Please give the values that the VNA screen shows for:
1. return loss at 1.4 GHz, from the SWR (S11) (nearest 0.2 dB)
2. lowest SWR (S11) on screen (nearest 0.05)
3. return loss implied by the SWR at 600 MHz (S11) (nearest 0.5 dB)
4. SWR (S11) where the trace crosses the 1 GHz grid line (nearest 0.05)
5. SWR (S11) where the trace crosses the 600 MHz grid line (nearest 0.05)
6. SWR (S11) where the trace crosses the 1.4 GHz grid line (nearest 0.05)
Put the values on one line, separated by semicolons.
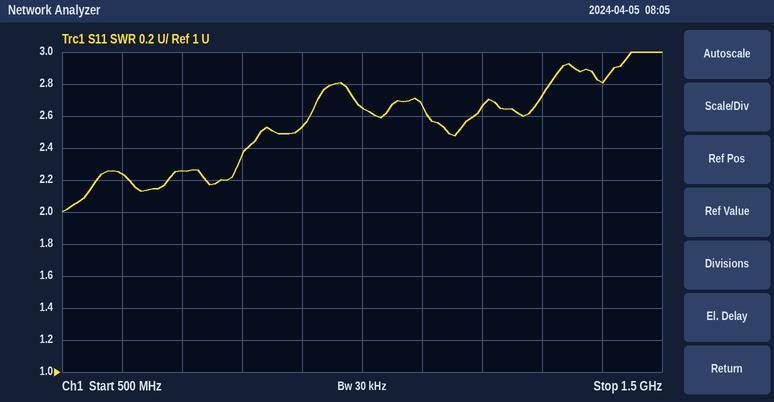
6.4 dB; 2.00; 8.5 dB; 2.65; 2.25; 2.80
